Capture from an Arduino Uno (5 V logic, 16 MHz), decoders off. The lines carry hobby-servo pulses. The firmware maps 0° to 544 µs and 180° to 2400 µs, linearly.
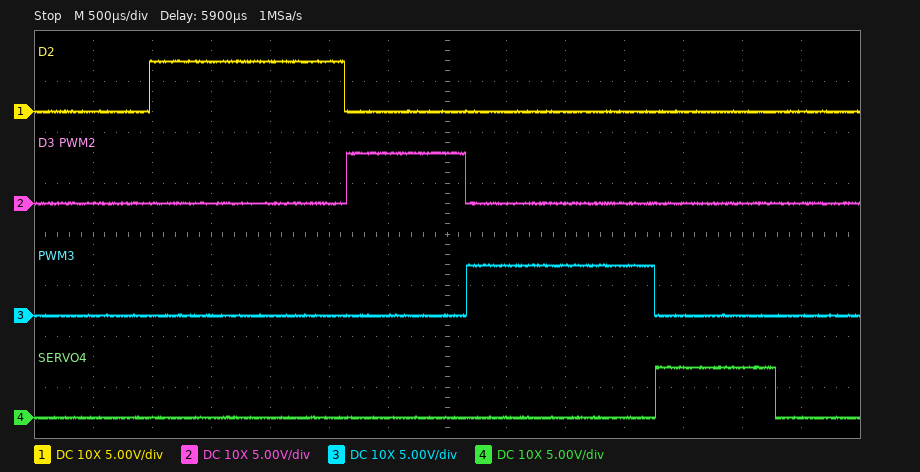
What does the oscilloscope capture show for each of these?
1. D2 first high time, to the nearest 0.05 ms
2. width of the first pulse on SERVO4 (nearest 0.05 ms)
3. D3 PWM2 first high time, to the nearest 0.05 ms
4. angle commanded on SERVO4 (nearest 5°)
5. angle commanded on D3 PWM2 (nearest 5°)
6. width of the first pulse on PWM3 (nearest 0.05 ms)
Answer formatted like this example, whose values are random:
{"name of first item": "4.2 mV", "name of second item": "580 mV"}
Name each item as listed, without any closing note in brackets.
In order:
{"D2 first high time, to the nearest 0.05 ms": "1.65 ms", "width of the first pulse on SERVO4": "1.00 ms", "D3 PWM2 first high time, to the nearest 0.05 ms": "1.00 ms", "angle commanded on SERVO4": "45°", "angle commanded on D3 PWM2": "45°", "width of the first pulse on PWM3": "1.60 ms"}
